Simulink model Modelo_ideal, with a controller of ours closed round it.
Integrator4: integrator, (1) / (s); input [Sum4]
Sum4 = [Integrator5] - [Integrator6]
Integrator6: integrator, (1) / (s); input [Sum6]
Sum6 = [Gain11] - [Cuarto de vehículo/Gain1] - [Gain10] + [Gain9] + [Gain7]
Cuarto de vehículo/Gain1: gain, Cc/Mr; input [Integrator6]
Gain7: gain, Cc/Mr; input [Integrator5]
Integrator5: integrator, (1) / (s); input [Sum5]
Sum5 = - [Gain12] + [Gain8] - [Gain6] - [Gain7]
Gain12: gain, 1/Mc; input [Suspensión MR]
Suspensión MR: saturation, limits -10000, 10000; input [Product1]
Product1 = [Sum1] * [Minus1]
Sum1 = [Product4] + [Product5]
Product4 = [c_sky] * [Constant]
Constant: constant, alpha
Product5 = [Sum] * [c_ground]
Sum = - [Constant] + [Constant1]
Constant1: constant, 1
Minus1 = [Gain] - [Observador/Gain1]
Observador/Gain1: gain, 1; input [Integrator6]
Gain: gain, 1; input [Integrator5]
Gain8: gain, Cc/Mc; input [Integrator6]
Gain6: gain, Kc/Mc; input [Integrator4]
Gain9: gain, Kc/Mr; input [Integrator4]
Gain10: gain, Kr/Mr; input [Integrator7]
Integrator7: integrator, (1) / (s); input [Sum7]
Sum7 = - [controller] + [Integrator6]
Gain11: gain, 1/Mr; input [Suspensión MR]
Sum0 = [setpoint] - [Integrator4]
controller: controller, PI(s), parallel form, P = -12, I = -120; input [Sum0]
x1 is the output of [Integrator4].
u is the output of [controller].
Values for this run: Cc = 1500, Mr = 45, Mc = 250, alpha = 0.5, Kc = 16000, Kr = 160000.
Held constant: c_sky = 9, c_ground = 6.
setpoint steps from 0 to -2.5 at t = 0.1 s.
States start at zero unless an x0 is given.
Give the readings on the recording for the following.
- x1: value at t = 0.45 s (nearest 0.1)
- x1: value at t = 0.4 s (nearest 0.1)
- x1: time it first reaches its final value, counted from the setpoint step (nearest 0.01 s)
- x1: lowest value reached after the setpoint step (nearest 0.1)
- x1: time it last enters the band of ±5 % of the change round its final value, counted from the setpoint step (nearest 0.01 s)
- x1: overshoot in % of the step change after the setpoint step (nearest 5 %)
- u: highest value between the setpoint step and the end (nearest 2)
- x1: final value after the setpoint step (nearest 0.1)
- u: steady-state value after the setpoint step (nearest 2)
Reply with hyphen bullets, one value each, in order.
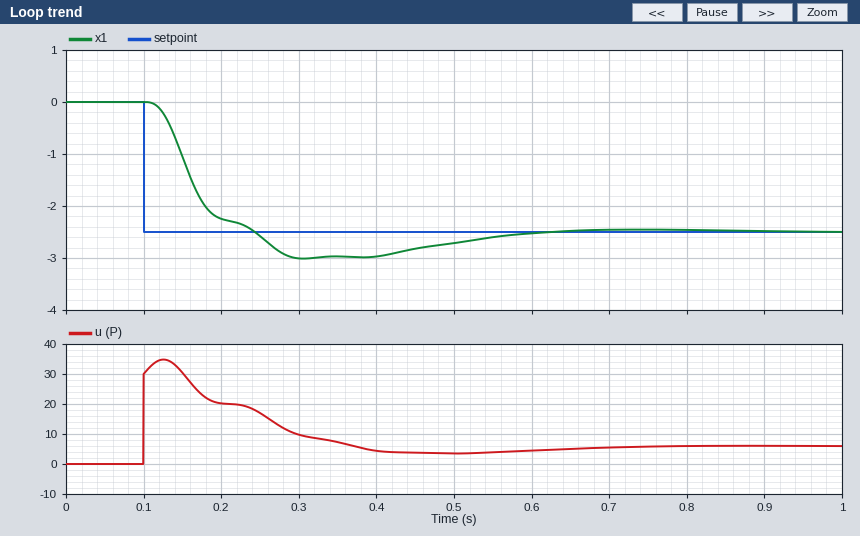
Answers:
- -2.8
- -3.0
- 0.14 s
- -3.0
- 0.44 s
- 20 %
- 34
- -2.5
- 6
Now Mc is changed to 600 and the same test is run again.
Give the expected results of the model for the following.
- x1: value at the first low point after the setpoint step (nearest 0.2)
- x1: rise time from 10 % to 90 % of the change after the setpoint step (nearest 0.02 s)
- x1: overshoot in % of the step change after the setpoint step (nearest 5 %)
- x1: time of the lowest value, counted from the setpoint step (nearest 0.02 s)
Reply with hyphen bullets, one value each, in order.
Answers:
- -3.2
- 0.06 s
- 30 %
- 0.20 s
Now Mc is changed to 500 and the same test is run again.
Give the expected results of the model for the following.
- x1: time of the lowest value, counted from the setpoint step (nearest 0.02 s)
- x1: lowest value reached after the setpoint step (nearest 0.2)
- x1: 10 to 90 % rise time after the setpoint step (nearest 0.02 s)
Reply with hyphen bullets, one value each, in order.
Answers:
- 0.20 s
- -3.2
- 0.06 s
